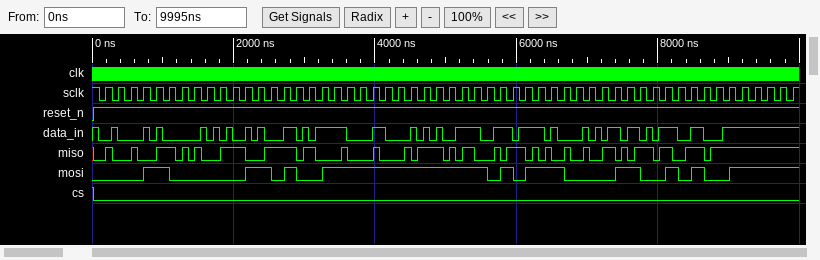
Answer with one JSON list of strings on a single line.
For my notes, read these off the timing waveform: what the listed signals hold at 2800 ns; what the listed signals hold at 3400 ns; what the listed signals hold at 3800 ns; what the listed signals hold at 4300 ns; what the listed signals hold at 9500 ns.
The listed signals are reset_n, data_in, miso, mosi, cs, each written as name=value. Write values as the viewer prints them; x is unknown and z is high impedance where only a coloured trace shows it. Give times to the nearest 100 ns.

["reset_n=1, data_in=1, miso=1, mosi=1, cs=0", "reset_n=1, data_in=1, miso=0, mosi=1, cs=0", "reset_n=1, data_in=0, miso=0, mosi=1, cs=0", "reset_n=1, data_in=0, miso=0, mosi=1, cs=0", "reset_n=1, data_in=1, miso=1, mosi=1, cs=0"]
